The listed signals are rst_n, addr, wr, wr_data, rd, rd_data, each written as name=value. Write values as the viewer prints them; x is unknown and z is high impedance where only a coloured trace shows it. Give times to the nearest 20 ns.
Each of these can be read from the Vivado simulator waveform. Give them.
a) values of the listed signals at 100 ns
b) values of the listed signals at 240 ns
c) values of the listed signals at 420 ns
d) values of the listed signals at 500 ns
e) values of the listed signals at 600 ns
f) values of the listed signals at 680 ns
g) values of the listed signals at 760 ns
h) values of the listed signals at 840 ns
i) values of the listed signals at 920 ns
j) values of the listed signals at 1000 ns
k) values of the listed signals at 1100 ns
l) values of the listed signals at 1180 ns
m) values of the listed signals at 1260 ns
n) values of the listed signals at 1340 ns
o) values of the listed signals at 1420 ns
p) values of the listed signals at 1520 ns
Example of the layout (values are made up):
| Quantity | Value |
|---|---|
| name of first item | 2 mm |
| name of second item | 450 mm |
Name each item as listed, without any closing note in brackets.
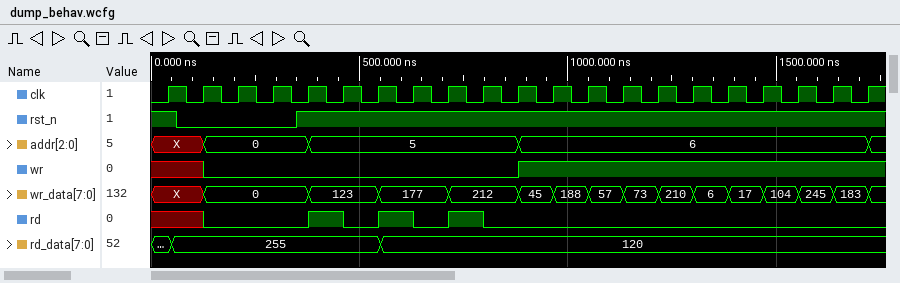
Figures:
| Quantity | Value |
|---|---|
| values of the listed signals at 100 ns | rst_n=0, addr=X, wr=x, wr_data=X, rd=x, rd_data=255 |
| values of the listed signals at 240 ns | rst_n=0, addr=0, wr=0, wr_data=0, rd=0, rd_data=255 |
| values of the listed signals at 420 ns | rst_n=1, addr=5, wr=0, wr_data=123, rd=1, rd_data=255 |
| values of the listed signals at 500 ns | rst_n=1, addr=5, wr=0, wr_data=123, rd=0, rd_data=255 |
| values of the listed signals at 600 ns | rst_n=1, addr=5, wr=0, wr_data=177, rd=1, rd_data=120 |
| values of the listed signals at 680 ns | rst_n=1, addr=5, wr=0, wr_data=177, rd=0, rd_data=120 |
| values of the listed signals at 760 ns | rst_n=1, addr=5, wr=0, wr_data=212, rd=1, rd_data=120 |
| values of the listed signals at 840 ns | rst_n=1, addr=5, wr=0, wr_data=212, rd=0, rd_data=120 |
| values of the listed signals at 920 ns | rst_n=1, addr=6, wr=1, wr_data=45, rd=0, rd_data=120 |
| values of the listed signals at 1000 ns | rst_n=1, addr=6, wr=1, wr_data=188, rd=0, rd_data=120 |
| values of the listed signals at 1100 ns | rst_n=1, addr=6, wr=1, wr_data=57, rd=0, rd_data=120 |
| values of the listed signals at 1180 ns | rst_n=1, addr=6, wr=1, wr_data=73, rd=0, rd_data=120 |
| values of the listed signals at 1260 ns | rst_n=1, addr=6, wr=1, wr_data=210, rd=0, rd_data=120 |
| values of the listed signals at 1340 ns | rst_n=1, addr=6, wr=1, wr_data=6, rd=0, rd_data=120 |
| values of the listed signals at 1420 ns | rst_n=1, addr=6, wr=1, wr_data=17, rd=0, rd_data=120 |
| values of the listed signals at 1520 ns | rst_n=1, addr=6, wr=1, wr_data=104, rd=0, rd_data=120 |
